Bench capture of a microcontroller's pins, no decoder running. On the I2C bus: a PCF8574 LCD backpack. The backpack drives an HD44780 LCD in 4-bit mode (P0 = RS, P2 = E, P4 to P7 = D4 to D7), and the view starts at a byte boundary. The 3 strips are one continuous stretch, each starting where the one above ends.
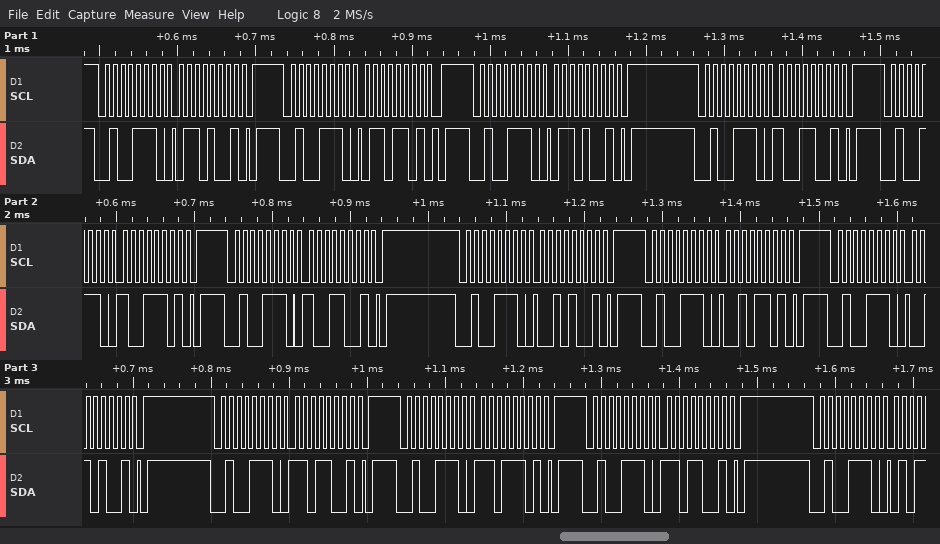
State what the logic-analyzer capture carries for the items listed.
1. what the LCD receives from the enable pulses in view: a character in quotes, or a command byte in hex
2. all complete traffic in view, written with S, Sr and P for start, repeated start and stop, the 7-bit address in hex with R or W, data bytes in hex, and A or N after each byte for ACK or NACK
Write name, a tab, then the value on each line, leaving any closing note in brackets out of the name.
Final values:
what the LCD receives from the enable pulses in view: a character in quotes, or a command byte in hex	'i' '-'
all complete traffic in view, written with S, Sr and P for start, repeated start and stop, the 7-bit address in hex with R or W, data bytes in hex, and A or N after each byte for ACK or NACK	S 27W A 69 A P S 27W A 6D A P S 27W A 69 A P S 27W A 99 A P S 27W A 9D A P S 27W A 99 A P S 27W A 29 A P S 27W A 2D A P S 27W A 29 A P S 27W A D9 A P S 27W A DD A P S 27W A D9 A P S 27W A
